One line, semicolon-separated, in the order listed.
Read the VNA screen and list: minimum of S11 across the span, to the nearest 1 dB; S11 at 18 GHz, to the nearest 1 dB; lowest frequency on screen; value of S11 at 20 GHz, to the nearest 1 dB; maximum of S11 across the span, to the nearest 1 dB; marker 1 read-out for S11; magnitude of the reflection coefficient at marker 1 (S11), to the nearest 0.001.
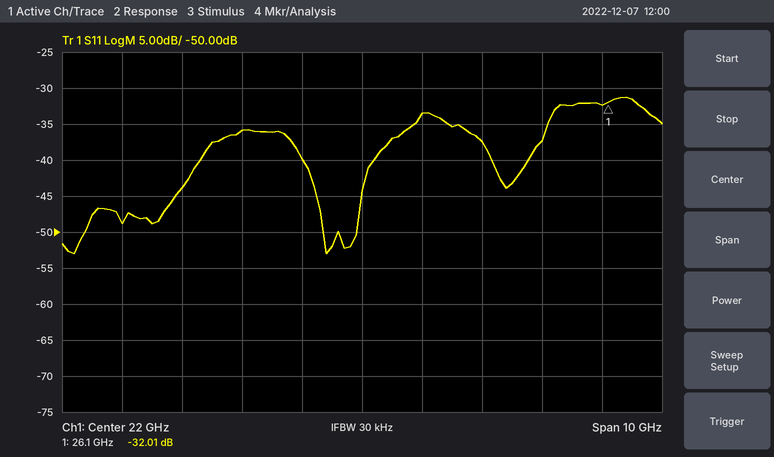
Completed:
-53 dB; -49 dB; 17 GHz; -36 dB; -31 dB; -32.01 dB; 0.025
